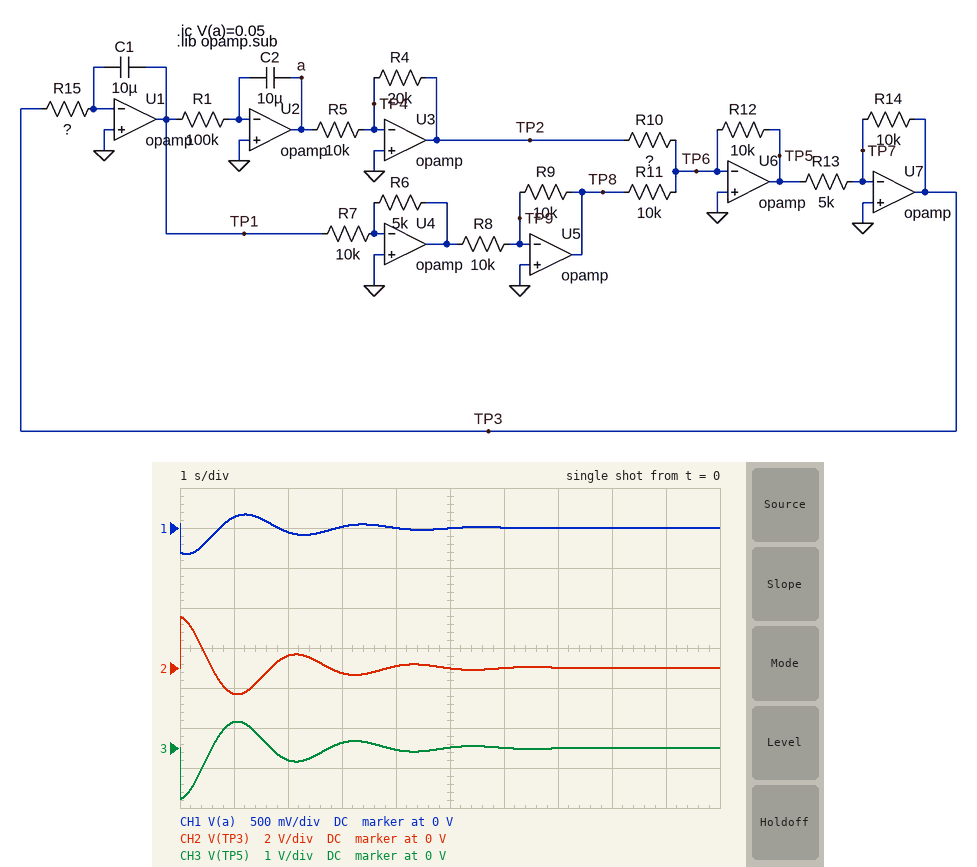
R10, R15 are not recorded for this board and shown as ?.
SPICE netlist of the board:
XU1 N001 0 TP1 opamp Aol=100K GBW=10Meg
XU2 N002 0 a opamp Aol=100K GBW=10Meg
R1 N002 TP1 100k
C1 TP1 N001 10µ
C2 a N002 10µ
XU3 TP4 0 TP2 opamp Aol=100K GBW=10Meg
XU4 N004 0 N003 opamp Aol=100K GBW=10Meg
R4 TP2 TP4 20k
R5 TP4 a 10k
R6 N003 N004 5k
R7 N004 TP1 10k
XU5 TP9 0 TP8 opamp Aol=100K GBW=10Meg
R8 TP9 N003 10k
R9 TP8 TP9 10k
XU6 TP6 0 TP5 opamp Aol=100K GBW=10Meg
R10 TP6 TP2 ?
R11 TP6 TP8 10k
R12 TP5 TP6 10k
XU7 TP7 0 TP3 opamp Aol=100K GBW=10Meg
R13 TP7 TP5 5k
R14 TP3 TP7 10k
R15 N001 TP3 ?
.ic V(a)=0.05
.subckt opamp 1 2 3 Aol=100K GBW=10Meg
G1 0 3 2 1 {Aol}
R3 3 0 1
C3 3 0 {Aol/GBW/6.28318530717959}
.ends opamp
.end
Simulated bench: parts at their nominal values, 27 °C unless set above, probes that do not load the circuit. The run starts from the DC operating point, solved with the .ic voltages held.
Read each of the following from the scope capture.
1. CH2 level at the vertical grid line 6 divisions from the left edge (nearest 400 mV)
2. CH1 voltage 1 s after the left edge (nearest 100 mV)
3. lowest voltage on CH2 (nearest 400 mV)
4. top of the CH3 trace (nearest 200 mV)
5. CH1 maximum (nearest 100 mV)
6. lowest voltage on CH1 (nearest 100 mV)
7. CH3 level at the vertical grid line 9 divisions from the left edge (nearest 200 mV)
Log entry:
0 V
100 mV
-1.2 V
600 mV
200 mV
-300 mV
0 V
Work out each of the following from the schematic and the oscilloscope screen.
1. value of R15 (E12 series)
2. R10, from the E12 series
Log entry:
82 kΩ
5.6 kΩ
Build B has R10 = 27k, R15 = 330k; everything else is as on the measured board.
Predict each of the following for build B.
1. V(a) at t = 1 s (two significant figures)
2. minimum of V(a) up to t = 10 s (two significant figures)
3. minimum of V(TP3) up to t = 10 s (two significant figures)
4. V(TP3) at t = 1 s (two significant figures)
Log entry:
-79 mV
-91 mV
-72 mV
150 mV
